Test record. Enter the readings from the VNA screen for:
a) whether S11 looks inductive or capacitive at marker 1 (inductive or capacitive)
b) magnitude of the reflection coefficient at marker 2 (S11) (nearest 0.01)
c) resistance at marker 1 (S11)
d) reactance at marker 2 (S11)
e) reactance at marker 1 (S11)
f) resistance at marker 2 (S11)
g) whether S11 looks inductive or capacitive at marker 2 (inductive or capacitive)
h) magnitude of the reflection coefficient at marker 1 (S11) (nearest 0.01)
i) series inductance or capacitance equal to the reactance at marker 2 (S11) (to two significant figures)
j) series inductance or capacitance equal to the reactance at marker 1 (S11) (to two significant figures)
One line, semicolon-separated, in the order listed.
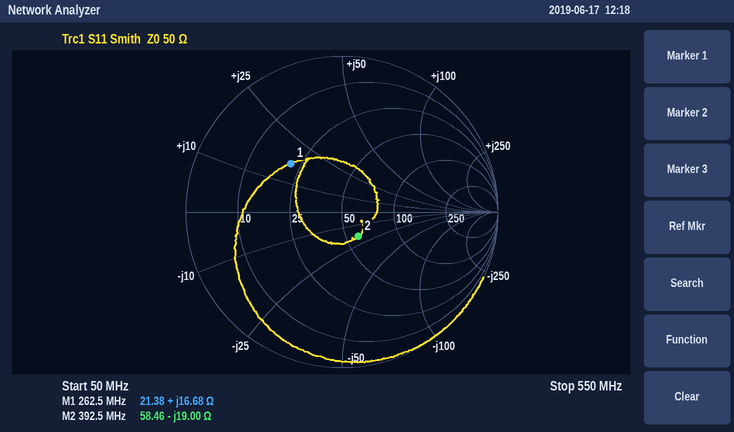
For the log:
inductive; 0.19; 21.38 Ω; -19.00 Ω; +16.68 Ω; 58.46 Ω; capacitive; 0.45; 21 pF; 10 nH
